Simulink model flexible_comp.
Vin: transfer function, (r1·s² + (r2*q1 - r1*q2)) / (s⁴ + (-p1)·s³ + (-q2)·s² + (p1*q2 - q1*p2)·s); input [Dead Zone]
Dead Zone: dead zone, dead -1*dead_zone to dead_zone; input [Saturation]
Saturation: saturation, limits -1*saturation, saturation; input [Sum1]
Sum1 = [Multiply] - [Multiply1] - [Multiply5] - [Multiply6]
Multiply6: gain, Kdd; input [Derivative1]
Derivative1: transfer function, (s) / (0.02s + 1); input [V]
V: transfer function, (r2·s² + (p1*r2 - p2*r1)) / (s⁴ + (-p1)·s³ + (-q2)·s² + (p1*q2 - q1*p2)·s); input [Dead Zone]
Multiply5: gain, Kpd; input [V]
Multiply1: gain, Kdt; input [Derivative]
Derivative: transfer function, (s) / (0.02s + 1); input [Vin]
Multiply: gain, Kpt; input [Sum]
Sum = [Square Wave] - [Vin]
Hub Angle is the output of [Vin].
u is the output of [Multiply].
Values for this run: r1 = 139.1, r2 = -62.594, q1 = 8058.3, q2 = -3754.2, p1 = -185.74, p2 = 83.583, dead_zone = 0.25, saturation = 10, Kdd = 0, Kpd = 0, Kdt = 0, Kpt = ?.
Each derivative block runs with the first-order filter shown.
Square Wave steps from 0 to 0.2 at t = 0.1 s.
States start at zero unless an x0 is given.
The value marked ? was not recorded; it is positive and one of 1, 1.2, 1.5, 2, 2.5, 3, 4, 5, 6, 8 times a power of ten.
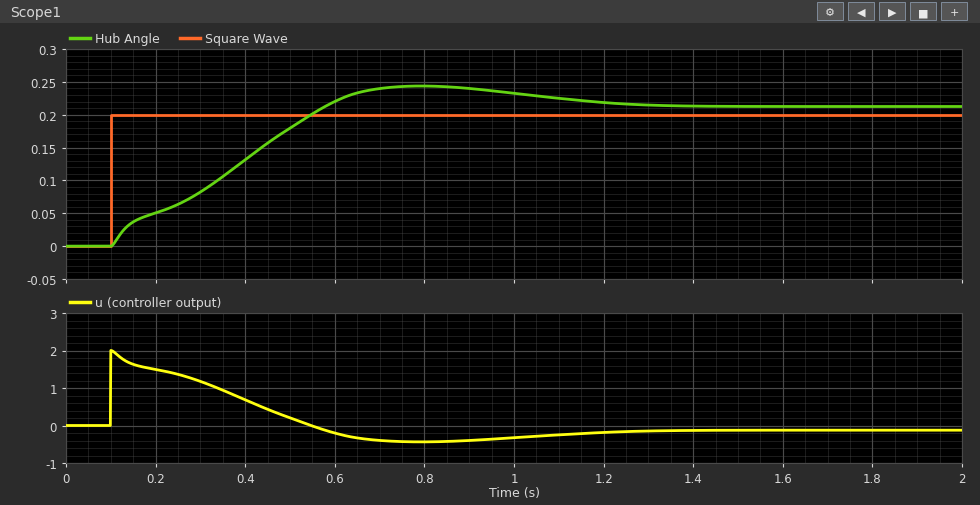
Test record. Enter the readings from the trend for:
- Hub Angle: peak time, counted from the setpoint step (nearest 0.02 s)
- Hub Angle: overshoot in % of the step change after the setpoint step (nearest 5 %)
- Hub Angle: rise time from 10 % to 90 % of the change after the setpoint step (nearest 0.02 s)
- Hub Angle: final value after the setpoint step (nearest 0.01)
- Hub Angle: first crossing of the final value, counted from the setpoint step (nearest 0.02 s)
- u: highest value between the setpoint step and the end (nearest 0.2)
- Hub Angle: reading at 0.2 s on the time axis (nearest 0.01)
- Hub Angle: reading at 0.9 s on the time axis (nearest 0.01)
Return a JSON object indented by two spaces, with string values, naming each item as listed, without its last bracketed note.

{
  "Hub Angle: peak time, counted from the setpoint step": "0.70 s",
  "Hub Angle: overshoot in % of the step change after the setpoint step": "15 %",
  "Hub Angle: rise time from 10 % to 90 % of the change after the setpoint step": "0.40 s",
  "Hub Angle: final value after the setpoint step": "0.21",
  "Hub Angle: first crossing of the final value, counted from the setpoint step": "0.48 s",
  "u: highest value between the setpoint step and the end": "2.0",
  "Hub Angle: reading at 0.2 s on the time axis": "0.05",
  "Hub Angle: reading at 0.9 s on the time axis": "0.24"
}
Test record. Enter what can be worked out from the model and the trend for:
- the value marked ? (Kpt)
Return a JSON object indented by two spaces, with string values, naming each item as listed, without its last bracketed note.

{
  "the value marked ?": "10"
}
